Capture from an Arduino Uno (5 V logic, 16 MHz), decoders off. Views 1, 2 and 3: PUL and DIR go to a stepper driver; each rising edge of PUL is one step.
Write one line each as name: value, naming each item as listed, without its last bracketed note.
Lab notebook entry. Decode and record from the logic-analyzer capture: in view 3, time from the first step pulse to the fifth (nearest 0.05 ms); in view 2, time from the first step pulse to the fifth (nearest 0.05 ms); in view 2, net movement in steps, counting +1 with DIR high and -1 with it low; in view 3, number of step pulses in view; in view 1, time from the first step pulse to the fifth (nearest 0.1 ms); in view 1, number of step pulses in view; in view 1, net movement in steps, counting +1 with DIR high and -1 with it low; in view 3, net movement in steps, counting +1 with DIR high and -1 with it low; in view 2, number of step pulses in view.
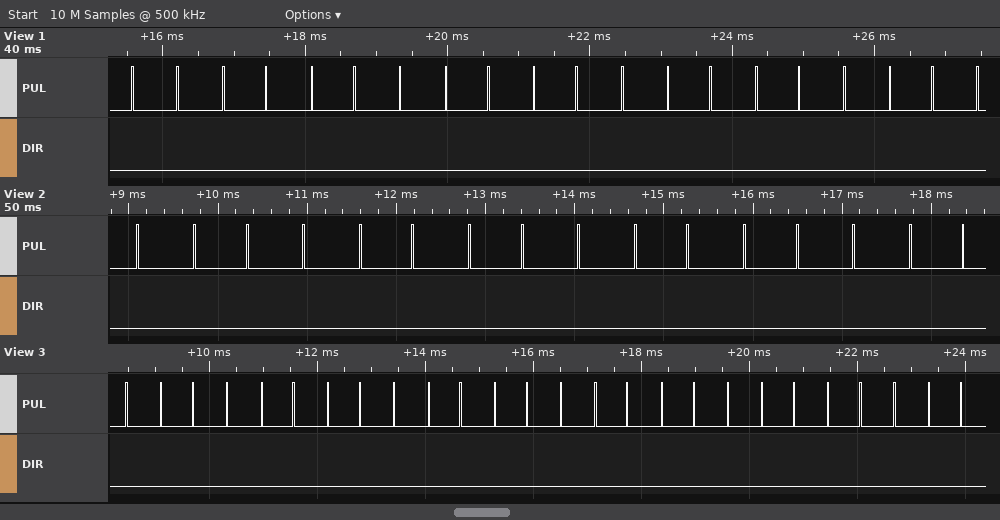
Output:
in view 3, time from the first step pulse to the fifth: 2.50 ms
in view 2, time from the first step pulse to the fifth: 2.50 ms
in view 2, net movement in steps, counting +1 with DIR high and -1 with it low: -16
in view 3, number of step pulses in view: 26
in view 1, time from the first step pulse to the fifth: 2.5 ms
in view 1, number of step pulses in view: 20
in view 1, net movement in steps, counting +1 with DIR high and -1 with it low: -20
in view 3, net movement in steps, counting +1 with DIR high and -1 with it low: -26
in view 2, number of step pulses in view: 16
